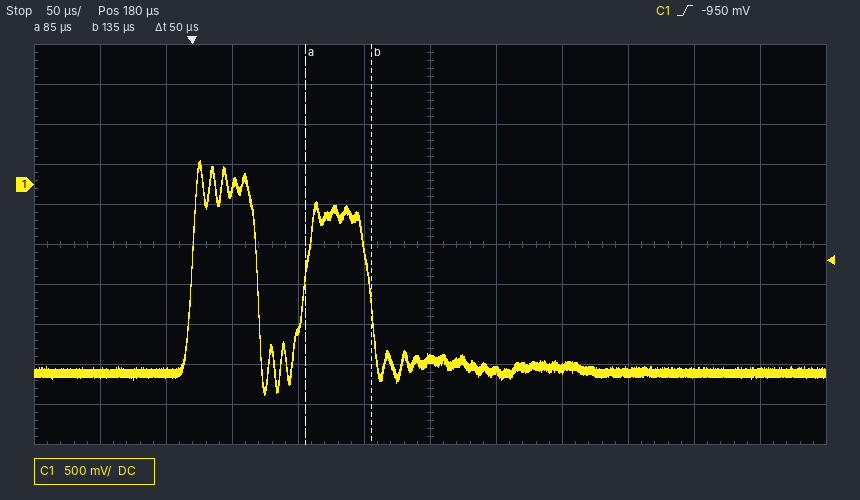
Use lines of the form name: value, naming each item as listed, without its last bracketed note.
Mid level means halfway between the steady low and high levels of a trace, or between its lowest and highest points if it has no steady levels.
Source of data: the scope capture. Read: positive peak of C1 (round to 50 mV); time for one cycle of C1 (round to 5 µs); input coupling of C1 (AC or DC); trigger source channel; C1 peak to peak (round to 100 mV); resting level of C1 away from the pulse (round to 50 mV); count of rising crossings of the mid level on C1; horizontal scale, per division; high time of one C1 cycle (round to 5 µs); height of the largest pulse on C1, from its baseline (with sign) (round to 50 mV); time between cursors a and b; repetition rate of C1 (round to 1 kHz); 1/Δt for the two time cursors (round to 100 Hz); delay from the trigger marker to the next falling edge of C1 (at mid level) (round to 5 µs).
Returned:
positive peak of C1: 300 mV
time for one cycle of C1: 85 µs
input coupling of C1: DC
trigger source channel: C1
C1 peak to peak: 2.90 V
resting level of C1 away from the pulse: -2.35 V
count of rising crossings of the mid level on C1: 2
horizontal scale, per division: 50 µs
high time of one C1 cycle: 50 µs
height of the largest pulse on C1, from its baseline (with sign): +2.65 V
time between cursors a and b: 50 µs
repetition rate of C1: 12 kHz
1/Δt for the two time cursors: 20.0 kHz
delay from the trigger marker to the next falling edge of C1 (at mid level): 50 µs
